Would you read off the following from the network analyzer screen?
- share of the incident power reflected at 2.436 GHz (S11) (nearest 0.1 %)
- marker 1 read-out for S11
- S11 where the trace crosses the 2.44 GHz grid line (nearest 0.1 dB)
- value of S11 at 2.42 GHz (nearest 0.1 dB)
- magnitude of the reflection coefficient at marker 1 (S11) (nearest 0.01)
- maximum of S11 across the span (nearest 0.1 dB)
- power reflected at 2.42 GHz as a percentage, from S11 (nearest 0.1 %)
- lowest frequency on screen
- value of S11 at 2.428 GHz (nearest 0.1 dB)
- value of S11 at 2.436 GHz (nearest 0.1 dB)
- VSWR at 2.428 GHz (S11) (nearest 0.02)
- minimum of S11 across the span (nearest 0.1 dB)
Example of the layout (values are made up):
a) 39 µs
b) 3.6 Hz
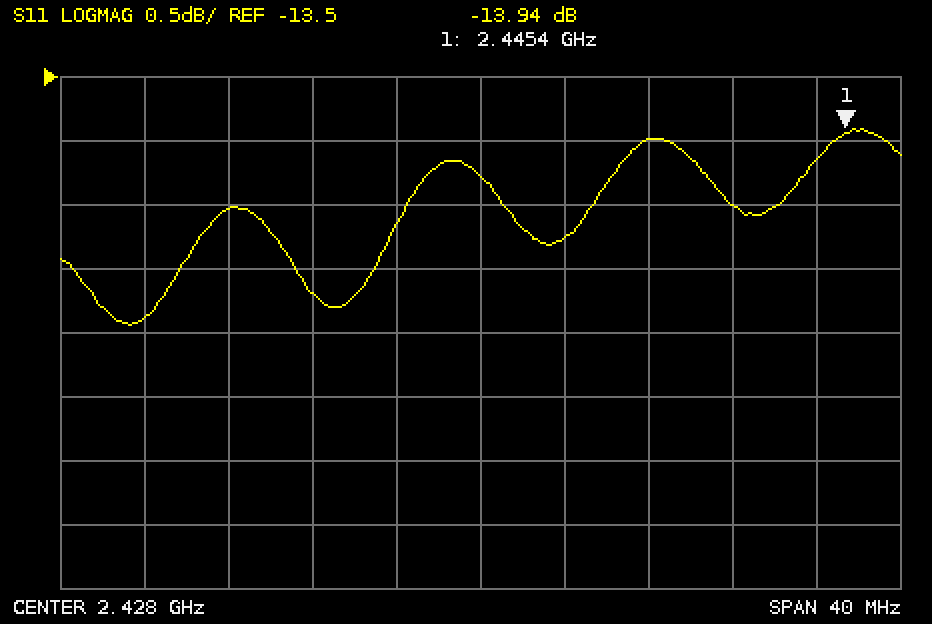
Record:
a) 4.0 %
b) -13.94 dB
c) -14.5 dB
d) -15.2 dB
e) 0.20
f) -13.9 dB
g) 3.0 %
h) 2.408 GHz
i) -14.3 dB
j) -14.0 dB
k) 1.48
l) -15.4 dB
